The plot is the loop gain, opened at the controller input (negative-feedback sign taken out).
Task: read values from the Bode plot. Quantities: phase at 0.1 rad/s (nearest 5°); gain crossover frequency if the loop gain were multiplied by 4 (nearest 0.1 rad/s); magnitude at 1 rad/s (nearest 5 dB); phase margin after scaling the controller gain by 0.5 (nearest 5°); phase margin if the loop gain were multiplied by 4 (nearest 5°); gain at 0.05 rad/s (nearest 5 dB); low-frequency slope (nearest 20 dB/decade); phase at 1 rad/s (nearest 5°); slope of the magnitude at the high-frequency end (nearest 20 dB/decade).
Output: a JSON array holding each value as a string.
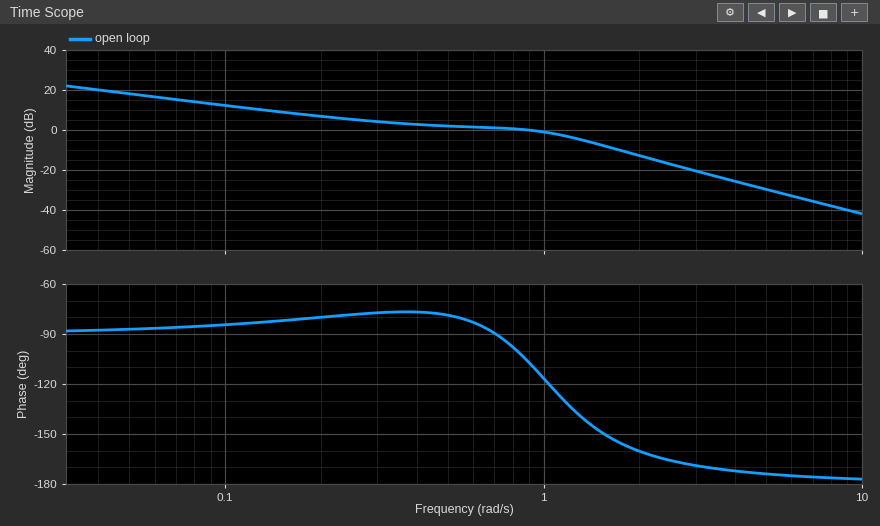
["-85°", "1.9 rad/s", "0 dB", "100°", "20°", "20 dB", "-20 dB/decade", "-115°", "-40 dB/decade"]
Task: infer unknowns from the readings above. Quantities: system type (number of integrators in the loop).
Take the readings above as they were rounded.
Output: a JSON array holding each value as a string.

["1"]
